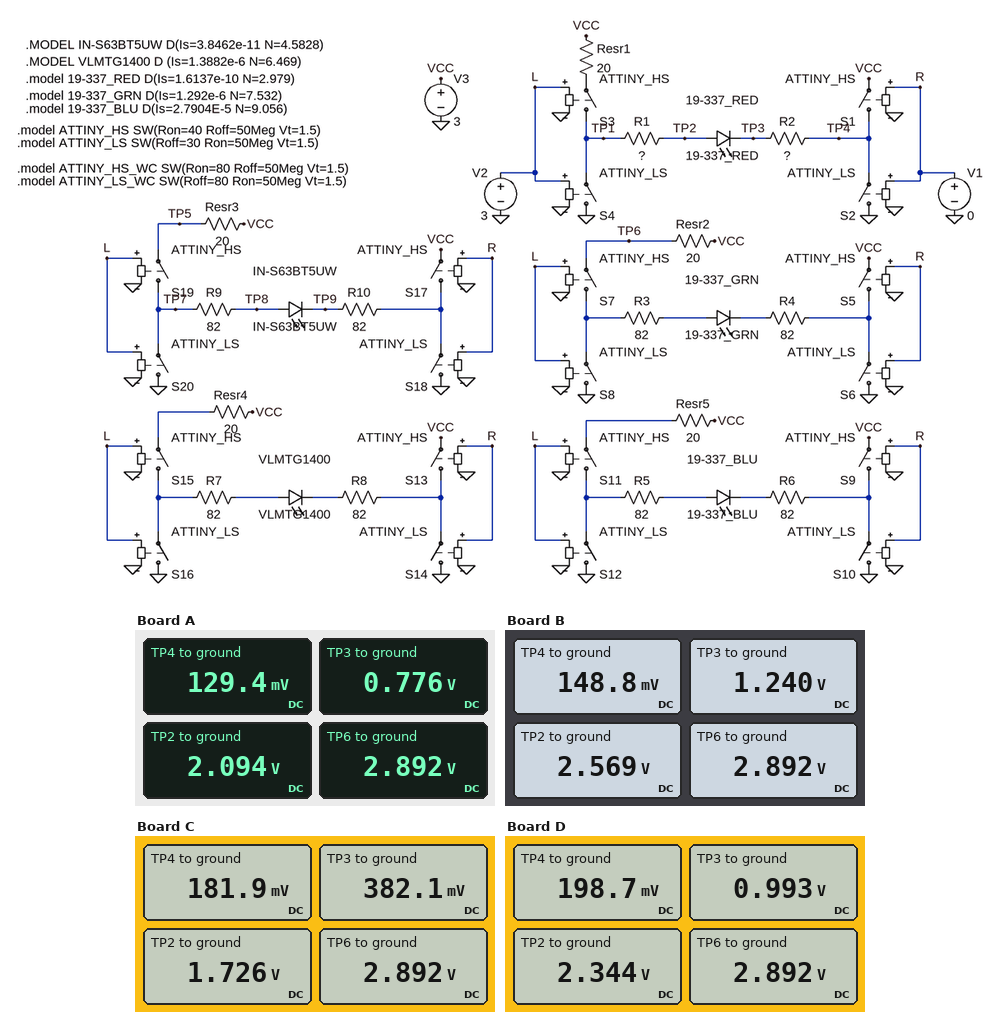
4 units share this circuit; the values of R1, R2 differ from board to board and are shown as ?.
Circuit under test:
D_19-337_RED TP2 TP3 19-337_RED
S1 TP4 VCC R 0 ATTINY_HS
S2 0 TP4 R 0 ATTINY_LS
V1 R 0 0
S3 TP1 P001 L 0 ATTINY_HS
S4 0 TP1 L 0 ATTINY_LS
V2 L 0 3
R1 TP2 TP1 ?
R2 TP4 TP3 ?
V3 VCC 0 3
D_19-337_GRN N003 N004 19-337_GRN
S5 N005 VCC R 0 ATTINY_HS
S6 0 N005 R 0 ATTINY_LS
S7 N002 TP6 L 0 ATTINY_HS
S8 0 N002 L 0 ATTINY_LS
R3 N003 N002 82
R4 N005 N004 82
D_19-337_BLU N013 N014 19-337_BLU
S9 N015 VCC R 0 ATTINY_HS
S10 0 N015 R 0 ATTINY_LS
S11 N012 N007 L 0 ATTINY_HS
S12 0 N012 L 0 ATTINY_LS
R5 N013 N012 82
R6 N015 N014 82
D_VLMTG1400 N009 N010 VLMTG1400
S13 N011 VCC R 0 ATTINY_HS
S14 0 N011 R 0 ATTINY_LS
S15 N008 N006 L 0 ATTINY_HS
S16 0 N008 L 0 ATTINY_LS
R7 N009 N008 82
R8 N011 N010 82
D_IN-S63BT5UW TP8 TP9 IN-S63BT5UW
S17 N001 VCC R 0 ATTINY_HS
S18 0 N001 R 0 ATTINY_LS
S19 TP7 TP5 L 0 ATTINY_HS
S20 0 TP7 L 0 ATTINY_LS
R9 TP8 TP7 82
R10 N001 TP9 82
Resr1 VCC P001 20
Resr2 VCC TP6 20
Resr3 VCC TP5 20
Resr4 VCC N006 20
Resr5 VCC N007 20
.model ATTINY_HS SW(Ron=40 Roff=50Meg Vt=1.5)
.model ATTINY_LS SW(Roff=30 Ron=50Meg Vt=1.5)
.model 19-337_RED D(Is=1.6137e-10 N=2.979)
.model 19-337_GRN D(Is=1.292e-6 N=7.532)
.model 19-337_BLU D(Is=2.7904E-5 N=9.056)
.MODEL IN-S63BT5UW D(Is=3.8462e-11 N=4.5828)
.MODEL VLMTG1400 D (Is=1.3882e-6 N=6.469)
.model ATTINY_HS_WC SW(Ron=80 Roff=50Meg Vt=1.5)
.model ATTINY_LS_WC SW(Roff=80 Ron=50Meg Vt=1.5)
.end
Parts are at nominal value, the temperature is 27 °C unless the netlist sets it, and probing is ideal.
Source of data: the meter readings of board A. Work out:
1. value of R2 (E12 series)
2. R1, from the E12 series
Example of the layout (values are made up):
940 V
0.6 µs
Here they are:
150 Ω
150 Ω
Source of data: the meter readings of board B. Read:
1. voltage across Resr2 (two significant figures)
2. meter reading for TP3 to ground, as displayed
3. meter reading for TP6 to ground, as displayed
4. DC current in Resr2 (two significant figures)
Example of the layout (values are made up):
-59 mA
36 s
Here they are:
110 mV
1.240 V
2.892 V
5.4 mA
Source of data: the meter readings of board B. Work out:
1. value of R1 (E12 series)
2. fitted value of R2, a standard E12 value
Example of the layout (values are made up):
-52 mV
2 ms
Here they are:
27 Ω
220 Ω
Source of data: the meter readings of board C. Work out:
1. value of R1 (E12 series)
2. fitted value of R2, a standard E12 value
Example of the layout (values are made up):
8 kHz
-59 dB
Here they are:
150 Ω
33 Ω
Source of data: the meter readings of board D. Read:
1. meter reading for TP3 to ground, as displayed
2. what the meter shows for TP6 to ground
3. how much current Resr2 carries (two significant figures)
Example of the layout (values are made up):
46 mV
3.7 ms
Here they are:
0.993 V
2.892 V
5.4 mA
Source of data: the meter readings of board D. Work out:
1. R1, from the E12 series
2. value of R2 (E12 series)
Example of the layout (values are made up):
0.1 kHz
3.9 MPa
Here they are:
39 Ω
120 Ω
